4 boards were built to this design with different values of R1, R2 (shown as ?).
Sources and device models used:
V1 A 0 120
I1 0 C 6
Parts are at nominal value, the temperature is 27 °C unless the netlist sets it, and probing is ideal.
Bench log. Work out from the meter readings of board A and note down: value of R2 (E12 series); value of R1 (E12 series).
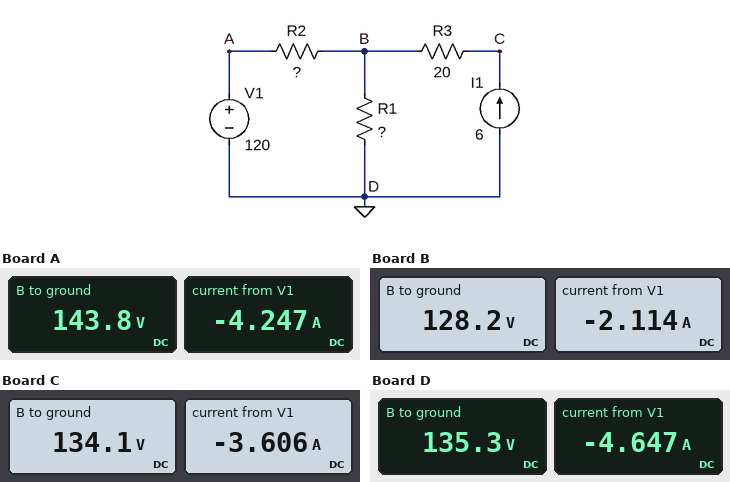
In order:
5.6 Ω
82 Ω
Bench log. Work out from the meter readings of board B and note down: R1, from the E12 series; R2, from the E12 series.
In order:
33 Ω
3.9 Ω
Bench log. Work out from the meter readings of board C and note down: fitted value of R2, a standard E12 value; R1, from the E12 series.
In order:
3.9 Ω
56 Ω
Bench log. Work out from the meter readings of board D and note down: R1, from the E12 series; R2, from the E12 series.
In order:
100 Ω
3.3 Ω
